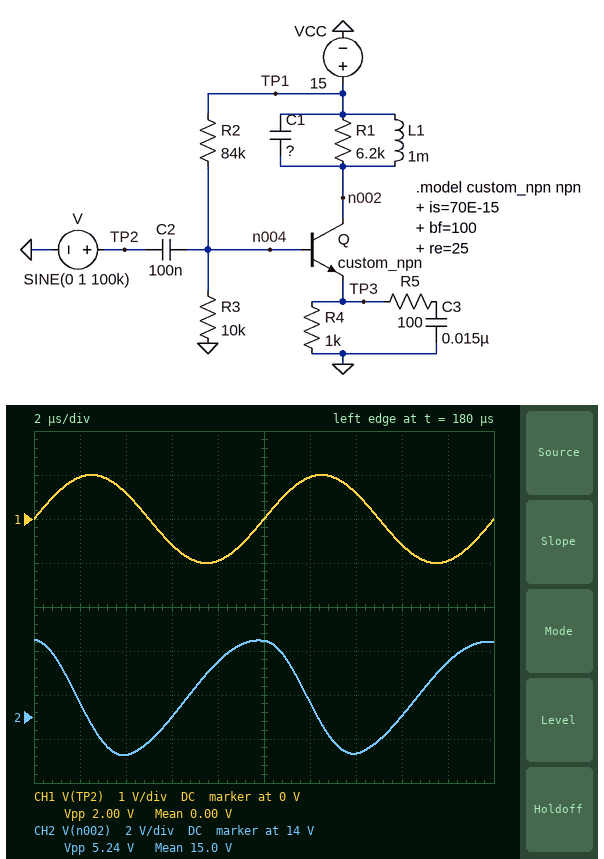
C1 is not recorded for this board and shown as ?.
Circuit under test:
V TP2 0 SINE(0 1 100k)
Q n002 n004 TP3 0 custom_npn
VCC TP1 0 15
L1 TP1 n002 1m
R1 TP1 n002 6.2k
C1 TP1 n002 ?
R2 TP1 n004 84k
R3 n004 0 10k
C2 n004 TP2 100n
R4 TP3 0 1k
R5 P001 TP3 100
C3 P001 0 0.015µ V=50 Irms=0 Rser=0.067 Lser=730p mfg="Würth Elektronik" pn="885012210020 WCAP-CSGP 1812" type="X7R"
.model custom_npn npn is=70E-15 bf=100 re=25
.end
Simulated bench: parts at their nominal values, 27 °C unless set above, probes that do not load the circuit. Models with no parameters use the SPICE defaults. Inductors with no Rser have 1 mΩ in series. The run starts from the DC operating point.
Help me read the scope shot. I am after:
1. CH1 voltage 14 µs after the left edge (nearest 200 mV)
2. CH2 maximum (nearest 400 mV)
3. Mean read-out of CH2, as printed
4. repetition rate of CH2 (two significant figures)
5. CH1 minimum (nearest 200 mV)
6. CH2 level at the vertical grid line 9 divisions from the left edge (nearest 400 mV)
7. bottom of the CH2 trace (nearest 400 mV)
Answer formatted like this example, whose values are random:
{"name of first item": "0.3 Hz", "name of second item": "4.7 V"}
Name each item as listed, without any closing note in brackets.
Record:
{"CH1 voltage 14 µs after the left edge": "600 mV", "CH2 maximum": "17.6 V", "Mean read-out of CH2, as printed": "15.0 V", "repetition rate of CH2": "100 kHz", "CH1 minimum": "-1.0 V", "CH2 level at the vertical grid line 9 divisions from the left edge": "16.4 V", "bottom of the CH2 trace": "12.4 V"}
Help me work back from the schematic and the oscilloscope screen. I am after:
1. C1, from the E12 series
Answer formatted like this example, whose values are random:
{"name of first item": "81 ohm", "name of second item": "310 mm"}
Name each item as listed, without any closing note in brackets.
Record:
{"C1, from the E12 series": "3.9 nF"}
